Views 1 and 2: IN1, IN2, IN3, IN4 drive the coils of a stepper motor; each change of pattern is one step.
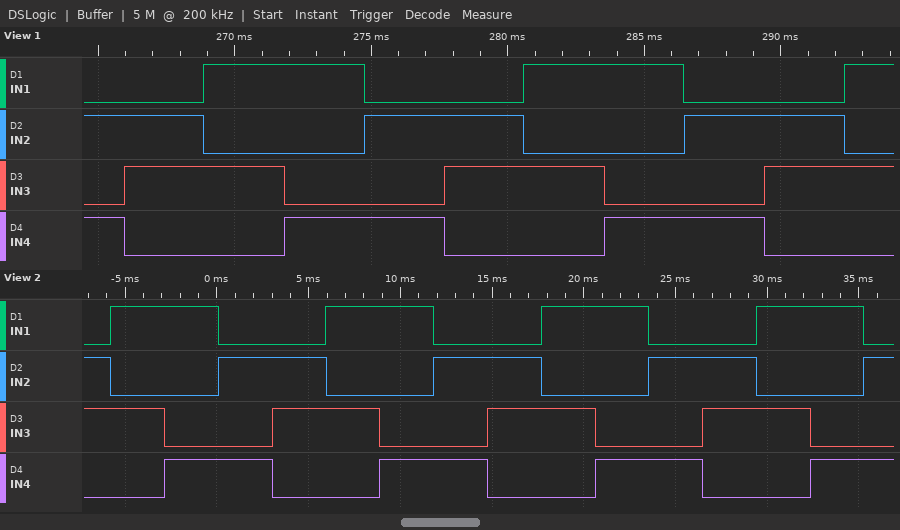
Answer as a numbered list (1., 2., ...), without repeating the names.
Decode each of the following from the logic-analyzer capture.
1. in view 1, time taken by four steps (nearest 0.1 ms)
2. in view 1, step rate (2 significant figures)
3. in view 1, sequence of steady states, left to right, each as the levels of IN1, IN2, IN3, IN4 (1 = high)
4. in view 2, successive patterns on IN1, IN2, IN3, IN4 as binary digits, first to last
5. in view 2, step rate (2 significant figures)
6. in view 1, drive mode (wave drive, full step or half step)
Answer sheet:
1. 11.7 ms
2. 340 steps/s
3. 0101 0110 1010 1001 0101 0110 1010 1001 0101 0110 1010
4. 0110 1010 1001 0101 0110 1010 1001 0101 0110 1010 1001 0101 0110 1010 1001 0101
5. 340 steps/s
6. full step
